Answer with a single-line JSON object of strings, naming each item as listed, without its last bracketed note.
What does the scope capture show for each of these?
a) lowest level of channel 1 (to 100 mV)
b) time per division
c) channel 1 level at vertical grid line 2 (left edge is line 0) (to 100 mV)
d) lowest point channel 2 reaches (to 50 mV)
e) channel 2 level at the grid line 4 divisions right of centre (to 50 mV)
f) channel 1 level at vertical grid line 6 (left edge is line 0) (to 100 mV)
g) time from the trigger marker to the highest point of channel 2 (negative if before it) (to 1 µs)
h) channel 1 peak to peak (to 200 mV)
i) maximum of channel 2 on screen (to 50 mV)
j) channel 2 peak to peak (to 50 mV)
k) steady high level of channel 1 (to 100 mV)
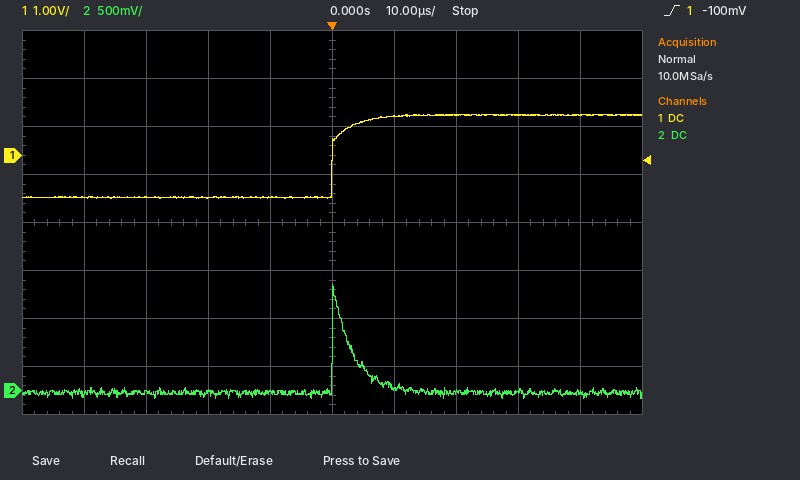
{"lowest level of channel 1": "-900 mV", "time per division": "10 µs", "channel 1 level at vertical grid line 2 (left edge is line 0)": "-900 mV", "lowest point channel 2 reaches": "-100 mV", "channel 2 level at the grid line 4 divisions right of centre": "0 mV", "channel 1 level at vertical grid line 6 (left edge is line 0)": "800 mV", "time from the trigger marker to the highest point of channel 2 (negative if before it)": "0 µs", "channel 1 peak to peak": "1.8 V", "maximum of channel 2 on screen": "1.10 V", "channel 2 peak to peak": "1.20 V", "steady high level of channel 1": "800 mV"}
